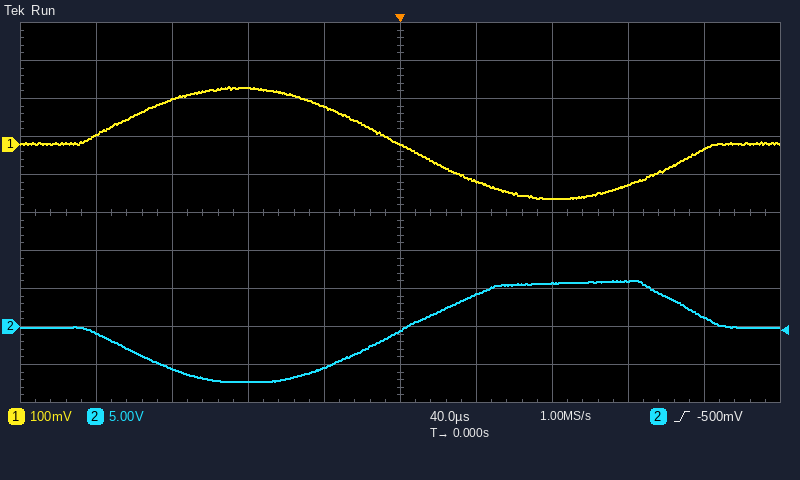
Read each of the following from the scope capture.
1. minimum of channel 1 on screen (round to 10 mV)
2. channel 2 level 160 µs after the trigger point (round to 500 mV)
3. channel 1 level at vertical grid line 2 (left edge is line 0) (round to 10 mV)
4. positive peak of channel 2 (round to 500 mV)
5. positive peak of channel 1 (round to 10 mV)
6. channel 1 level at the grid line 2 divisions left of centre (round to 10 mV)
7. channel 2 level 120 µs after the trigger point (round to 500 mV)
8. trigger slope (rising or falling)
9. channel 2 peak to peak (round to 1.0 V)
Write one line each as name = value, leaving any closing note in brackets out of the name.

minimum of channel 1 on screen = -140 mV
channel 2 level 160 µs after the trigger point = 1.0 V
channel 1 level at vertical grid line 2 (left edge is line 0) = 120 mV
positive peak of channel 2 = 6.0 V
positive peak of channel 1 = 150 mV
channel 1 level at the grid line 2 divisions left of centre = 150 mV
channel 2 level 120 µs after the trigger point = 6.0 V
trigger slope = rising
channel 2 peak to peak = 13.0 V
